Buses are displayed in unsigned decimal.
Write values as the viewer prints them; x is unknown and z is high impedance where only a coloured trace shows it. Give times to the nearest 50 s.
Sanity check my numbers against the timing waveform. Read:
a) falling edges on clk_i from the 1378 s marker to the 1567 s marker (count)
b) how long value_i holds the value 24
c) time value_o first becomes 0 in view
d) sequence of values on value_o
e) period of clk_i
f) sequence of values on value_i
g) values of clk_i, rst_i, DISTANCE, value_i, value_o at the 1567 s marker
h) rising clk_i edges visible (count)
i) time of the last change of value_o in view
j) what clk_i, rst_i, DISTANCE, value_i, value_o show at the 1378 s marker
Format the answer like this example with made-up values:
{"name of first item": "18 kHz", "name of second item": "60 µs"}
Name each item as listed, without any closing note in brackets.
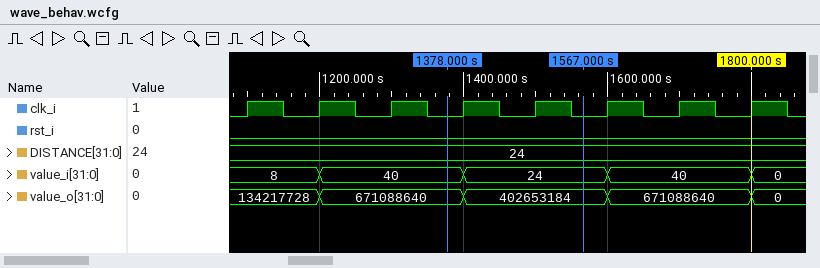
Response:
{"falling edges on clk_i from the 1378 s marker to the 1567 s marker": "2", "how long value_i holds the value 24": "200 s", "time value_o first becomes 0 in view": "1800 s", "sequence of values on value_o": "134217728, 671088640, 402653184, 671088640, 0", "period of clk_i": "100 s", "sequence of values on value_i": "8, 40, 24, 40, 0", "values of clk_i, rst_i, DISTANCE, value_i, value_o at the 1567 s marker": "clk_i=0, rst_i=0, DISTANCE=24, value_i=24, value_o=402653184", "rising clk_i edges visible": "8", "time of the last change of value_o in view": "1800 s", "what clk_i, rst_i, DISTANCE, value_i, value_o show at the 1378 s marker": "clk_i=0, rst_i=0, DISTANCE=24, value_i=40, value_o=671088640"}
